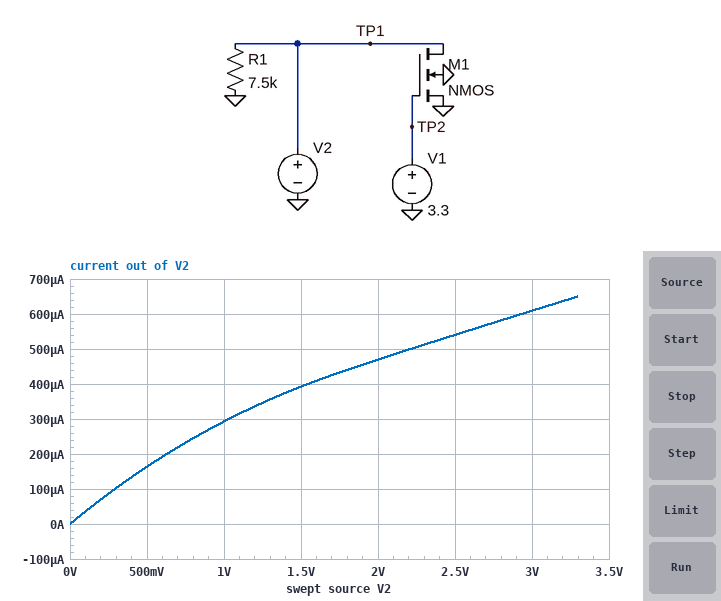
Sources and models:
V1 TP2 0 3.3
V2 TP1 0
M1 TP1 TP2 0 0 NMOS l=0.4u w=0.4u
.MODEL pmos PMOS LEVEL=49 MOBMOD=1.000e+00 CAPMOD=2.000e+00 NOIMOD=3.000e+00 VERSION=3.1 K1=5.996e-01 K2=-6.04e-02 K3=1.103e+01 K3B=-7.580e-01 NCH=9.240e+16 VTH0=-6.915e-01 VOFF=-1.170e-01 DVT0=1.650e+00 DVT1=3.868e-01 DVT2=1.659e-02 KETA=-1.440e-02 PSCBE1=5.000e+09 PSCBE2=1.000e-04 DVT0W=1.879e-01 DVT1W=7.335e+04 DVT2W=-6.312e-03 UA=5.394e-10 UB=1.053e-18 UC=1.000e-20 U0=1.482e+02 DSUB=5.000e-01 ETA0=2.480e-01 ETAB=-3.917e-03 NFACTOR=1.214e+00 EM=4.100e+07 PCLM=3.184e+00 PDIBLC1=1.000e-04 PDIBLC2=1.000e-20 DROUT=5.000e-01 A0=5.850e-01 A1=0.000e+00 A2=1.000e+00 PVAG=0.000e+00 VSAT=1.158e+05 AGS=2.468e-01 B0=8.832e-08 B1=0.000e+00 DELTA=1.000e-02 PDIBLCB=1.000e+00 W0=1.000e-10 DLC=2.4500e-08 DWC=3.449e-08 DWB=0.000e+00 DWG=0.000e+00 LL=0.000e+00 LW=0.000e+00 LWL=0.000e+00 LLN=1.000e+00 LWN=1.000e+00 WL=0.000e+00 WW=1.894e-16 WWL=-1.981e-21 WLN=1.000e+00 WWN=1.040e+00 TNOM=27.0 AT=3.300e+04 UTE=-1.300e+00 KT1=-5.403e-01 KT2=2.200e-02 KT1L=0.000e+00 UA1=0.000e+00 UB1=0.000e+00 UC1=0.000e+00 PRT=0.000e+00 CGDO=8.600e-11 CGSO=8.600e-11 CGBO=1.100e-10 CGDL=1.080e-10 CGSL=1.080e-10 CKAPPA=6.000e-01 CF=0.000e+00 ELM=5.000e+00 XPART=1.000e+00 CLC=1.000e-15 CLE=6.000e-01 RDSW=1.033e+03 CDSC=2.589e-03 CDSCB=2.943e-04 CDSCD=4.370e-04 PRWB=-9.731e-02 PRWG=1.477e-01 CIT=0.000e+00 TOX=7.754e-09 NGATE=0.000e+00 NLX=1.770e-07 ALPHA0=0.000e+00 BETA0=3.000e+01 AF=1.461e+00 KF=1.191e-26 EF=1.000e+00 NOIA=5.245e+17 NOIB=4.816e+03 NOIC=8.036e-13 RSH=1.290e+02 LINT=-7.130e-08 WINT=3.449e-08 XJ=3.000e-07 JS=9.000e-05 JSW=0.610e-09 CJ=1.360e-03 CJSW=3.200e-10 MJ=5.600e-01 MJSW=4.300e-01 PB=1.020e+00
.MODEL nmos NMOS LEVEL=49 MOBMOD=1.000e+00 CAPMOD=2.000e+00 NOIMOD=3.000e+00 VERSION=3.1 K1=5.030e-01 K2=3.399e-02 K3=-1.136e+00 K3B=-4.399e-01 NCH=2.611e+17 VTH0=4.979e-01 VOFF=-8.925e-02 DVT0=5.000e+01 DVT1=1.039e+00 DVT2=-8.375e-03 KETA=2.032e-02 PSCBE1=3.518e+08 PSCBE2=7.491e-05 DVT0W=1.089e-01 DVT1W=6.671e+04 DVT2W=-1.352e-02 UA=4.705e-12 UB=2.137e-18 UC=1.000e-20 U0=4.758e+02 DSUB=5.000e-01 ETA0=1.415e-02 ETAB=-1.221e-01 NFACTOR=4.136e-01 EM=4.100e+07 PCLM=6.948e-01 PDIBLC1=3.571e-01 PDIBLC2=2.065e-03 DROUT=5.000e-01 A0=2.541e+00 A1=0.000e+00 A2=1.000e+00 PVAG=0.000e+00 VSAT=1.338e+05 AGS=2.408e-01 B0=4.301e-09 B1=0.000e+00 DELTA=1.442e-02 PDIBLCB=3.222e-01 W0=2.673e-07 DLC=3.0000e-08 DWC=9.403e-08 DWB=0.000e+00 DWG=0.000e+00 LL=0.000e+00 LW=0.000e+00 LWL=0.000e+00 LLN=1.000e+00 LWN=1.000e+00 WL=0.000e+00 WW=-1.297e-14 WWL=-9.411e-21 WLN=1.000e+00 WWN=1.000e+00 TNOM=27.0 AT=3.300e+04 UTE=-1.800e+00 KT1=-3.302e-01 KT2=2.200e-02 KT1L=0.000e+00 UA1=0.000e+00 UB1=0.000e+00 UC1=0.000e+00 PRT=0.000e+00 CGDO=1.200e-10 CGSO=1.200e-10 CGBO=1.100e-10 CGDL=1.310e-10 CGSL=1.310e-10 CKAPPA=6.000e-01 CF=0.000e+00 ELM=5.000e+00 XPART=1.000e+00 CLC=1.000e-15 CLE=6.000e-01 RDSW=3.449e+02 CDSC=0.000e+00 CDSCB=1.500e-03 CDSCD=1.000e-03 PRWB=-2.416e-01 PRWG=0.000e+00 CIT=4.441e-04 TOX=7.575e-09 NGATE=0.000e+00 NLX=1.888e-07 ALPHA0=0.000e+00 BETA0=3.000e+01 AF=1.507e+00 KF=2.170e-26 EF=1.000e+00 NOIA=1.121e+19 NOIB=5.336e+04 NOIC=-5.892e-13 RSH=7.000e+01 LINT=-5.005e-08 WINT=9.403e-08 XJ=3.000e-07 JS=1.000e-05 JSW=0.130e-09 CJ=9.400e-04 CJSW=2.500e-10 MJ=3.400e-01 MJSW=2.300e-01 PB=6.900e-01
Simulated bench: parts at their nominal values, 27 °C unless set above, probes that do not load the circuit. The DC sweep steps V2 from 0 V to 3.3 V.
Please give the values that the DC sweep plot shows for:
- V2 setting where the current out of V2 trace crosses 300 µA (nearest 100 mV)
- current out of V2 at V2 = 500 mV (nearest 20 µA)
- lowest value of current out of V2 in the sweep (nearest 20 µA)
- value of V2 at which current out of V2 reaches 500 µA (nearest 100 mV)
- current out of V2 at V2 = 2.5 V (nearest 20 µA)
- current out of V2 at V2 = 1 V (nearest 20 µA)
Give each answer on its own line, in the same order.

1.0 V
160 µA
0 A
2.2 V
540 µA
300 µA
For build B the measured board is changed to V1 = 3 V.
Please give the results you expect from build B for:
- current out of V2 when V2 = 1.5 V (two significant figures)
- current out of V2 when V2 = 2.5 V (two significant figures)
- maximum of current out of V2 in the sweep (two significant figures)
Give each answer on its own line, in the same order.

370 µA
510 µA
620 µA
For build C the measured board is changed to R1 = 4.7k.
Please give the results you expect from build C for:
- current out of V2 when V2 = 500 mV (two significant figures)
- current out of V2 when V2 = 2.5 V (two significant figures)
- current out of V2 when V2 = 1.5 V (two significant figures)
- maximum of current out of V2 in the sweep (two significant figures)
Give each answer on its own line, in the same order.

200 µA
740 µA
510 µA
910 µA
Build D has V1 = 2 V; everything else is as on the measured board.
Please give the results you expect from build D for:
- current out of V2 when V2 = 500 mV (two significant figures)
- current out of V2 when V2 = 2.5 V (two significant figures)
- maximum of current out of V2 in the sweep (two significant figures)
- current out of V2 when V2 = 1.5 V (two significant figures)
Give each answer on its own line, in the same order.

130 µA
420 µA
530 µA
280 µA
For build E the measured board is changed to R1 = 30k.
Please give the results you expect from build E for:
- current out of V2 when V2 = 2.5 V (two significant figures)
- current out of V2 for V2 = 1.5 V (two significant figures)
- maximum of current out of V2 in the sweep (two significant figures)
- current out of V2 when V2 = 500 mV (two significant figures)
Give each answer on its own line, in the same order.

290 µA
240 µA
320 µA
110 µA
